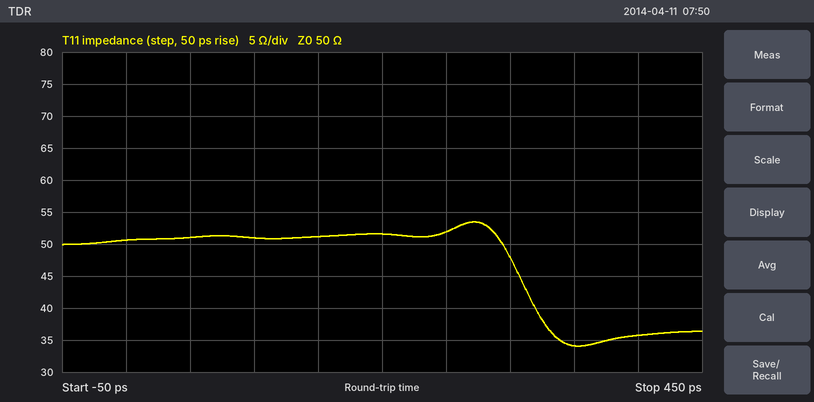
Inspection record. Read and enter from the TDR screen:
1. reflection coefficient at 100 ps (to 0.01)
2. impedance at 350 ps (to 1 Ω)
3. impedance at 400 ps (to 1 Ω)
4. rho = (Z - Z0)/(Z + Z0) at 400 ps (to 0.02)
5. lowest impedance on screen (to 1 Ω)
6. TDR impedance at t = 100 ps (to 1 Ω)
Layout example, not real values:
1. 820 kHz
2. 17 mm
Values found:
1. +0.01
2. 34 Ω
3. 36 Ω
4. -0.16
5. 34 Ω
6. 51 Ω
